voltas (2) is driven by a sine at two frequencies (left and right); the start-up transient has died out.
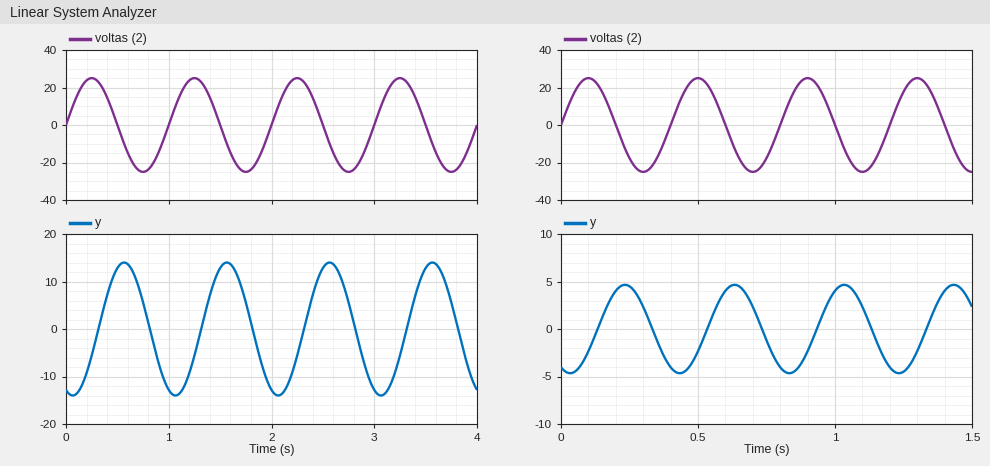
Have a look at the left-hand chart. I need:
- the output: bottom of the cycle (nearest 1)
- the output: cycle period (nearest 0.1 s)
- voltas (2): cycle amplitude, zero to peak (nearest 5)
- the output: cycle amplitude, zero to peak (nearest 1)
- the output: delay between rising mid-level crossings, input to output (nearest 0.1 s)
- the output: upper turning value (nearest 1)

-14
1.0 s
25
14
0.3 s
14
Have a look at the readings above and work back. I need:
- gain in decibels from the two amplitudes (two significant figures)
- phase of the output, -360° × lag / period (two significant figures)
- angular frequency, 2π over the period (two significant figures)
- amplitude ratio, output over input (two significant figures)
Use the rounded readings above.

-5.0 dB
-110°
6.3 rad/s
0.56
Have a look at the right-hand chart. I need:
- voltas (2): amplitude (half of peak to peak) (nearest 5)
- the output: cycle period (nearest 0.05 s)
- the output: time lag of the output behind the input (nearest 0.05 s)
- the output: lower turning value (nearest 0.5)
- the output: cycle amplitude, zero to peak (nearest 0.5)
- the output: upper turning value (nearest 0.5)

25
0.40 s
0.15 s
-4.5
4.5
4.5
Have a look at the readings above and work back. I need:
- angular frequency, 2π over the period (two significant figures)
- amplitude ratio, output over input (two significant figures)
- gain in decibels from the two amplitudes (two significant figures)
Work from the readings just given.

16 rad/s
0.18
-15 dB
